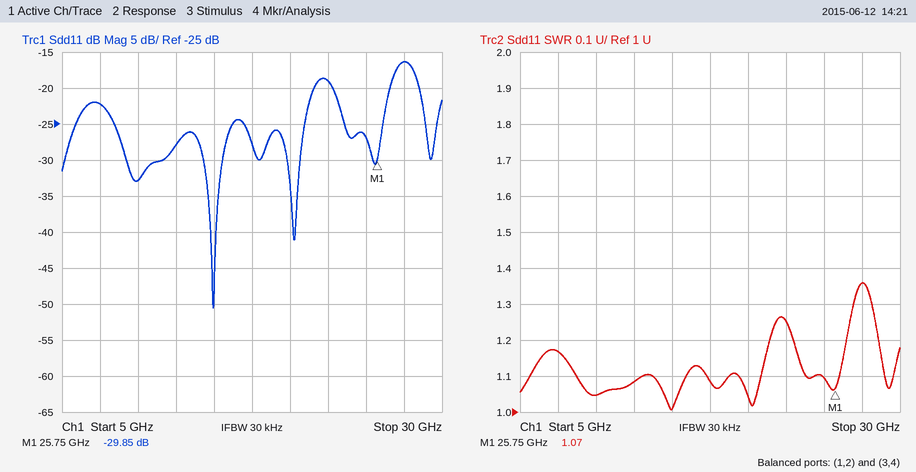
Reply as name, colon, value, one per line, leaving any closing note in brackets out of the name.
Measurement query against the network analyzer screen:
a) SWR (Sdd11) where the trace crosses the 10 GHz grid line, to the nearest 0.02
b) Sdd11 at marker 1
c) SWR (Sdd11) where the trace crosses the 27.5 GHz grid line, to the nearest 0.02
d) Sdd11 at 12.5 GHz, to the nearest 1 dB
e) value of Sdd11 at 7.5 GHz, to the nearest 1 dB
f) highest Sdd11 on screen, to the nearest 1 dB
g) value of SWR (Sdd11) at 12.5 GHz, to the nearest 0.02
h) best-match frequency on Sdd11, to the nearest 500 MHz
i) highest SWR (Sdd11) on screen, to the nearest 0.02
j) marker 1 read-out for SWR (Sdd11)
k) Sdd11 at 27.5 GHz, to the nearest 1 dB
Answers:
SWR (Sdd11) where the trace crosses the 10 GHz grid line, to the nearest 0.02: 1.04
Sdd11 at marker 1: -29.85 dB
SWR (Sdd11) where the trace crosses the 27.5 GHz grid line, to the nearest 0.02: 1.36
Sdd11 at 12.5 GHz, to the nearest 1 dB: -28 dB
value of Sdd11 at 7.5 GHz, to the nearest 1 dB: -22 dB
highest Sdd11 on screen, to the nearest 1 dB: -16 dB
value of SWR (Sdd11) at 12.5 GHz, to the nearest 0.02: 1.08
best-match frequency on Sdd11, to the nearest 500 MHz: 15.0 GHz
highest SWR (Sdd11) on screen, to the nearest 0.02: 1.36
marker 1 read-out for SWR: 1.07
Sdd11 at 27.5 GHz, to the nearest 1 dB: -16 dB
